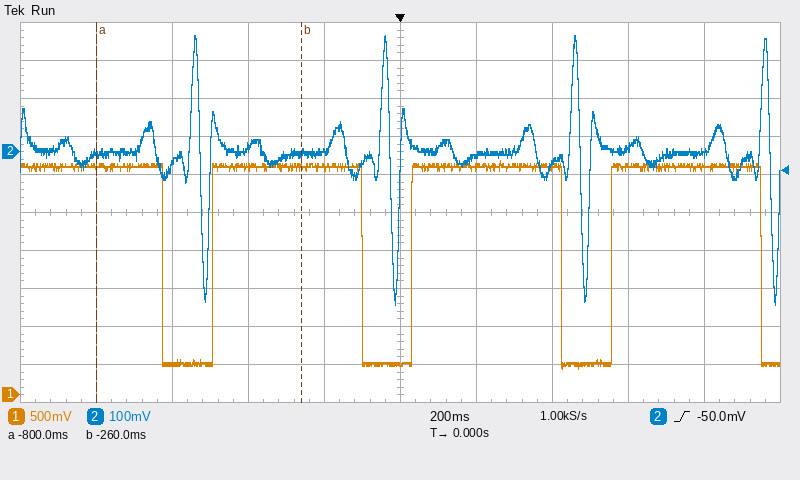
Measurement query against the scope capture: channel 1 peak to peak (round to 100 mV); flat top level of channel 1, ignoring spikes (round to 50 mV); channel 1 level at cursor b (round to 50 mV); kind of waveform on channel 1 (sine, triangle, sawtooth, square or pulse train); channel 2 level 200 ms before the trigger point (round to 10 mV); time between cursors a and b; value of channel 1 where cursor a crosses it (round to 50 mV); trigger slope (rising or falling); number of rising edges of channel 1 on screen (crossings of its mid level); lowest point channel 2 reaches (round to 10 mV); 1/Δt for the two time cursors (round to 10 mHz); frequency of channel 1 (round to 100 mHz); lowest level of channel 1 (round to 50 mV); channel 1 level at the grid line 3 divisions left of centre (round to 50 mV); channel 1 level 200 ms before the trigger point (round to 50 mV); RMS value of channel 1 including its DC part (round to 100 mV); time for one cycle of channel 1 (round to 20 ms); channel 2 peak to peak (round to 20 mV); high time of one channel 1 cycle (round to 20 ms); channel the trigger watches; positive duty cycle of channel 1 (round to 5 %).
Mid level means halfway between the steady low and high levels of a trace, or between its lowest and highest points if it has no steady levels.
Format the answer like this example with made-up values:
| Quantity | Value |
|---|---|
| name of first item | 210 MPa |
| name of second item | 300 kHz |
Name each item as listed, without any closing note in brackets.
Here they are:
| Quantity | Value |
|---|---|
| channel 1 peak to peak | 2.70 V |
| flat top level of channel 1, ignoring spikes | 3.00 V |
| channel 1 level at cursor b | 3.00 V |
| kind of waveform on channel 1 | pulse train |
| channel 2 level 200 ms before the trigger point | 0 mV |
| time between cursors a and b | 540 ms |
| value of channel 1 where cursor a crosses it | 3.00 V |
| trigger slope | rising |
| number of rising edges of channel 1 on screen | 3 |
| lowest point channel 2 reaches | -400 mV |
| 1/Δt for the two time cursors | 1.85 Hz |
| frequency of channel 1 | 1.9 Hz |
| lowest level of channel 1 | 350 mV |
| channel 1 level at the grid line 3 divisions left of centre | 400 mV |
| channel 1 level 200 ms before the trigger point | 3.00 V |
| RMS value of channel 1 including its DC part | 2.6 V |
| time for one cycle of channel 1 | 520 ms |
| channel 2 peak to peak | 700 mV |
| high time of one channel 1 cycle | 400 ms |
| channel the trigger watches | channel 2 |
| positive duty cycle of channel 1 | 75 % |
